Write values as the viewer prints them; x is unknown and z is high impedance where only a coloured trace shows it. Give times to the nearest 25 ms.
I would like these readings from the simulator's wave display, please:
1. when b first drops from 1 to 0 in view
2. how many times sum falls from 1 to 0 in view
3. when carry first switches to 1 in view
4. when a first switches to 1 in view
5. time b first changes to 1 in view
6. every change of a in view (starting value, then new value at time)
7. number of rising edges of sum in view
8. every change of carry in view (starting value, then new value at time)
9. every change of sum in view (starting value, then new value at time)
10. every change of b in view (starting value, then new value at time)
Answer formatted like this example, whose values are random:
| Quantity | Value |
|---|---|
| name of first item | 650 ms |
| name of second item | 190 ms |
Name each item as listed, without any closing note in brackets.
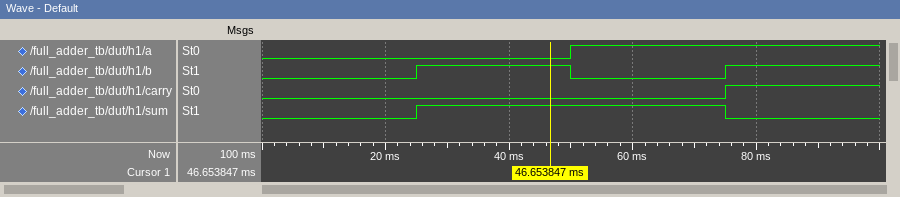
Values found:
| Quantity | Value |
|---|---|
| when b first drops from 1 to 0 in view | 50 ms |
| how many times sum falls from 1 to 0 in view | 1 |
| when carry first switches to 1 in view | 75 ms |
| when a first switches to 1 in view | 50 ms |
| time b first changes to 1 in view | 25 ms |
| every change of a in view | 0, 1 at 50 ms |
| number of rising edges of sum in view | 1 |
| every change of carry in view | 0, 1 at 75 ms |
| every change of sum in view | 0, 1 at 25 ms, 0 at 75 ms |
| every change of b in view | 0, 1 at 25 ms, 0 at 50 ms, 1 at 75 ms |
